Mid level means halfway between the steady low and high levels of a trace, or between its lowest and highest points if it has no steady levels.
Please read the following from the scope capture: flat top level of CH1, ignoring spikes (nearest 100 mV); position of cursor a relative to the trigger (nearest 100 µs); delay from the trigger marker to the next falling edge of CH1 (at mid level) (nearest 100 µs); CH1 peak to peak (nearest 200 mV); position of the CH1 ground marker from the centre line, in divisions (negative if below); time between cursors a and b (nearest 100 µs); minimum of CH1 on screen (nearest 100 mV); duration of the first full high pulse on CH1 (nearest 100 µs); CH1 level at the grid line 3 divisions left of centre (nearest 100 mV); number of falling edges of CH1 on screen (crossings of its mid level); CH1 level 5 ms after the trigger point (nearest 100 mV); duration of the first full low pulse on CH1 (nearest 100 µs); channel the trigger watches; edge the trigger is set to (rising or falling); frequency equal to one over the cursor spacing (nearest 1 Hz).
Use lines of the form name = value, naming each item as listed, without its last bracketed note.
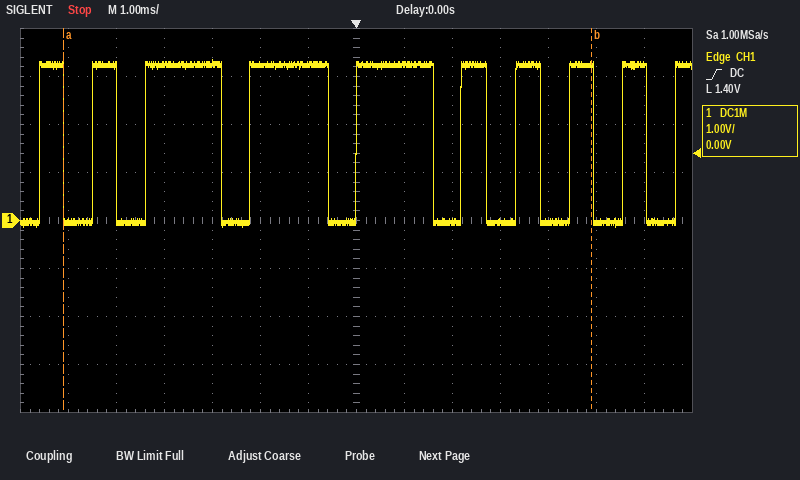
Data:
flat top level of CH1, ignoring spikes = 3.2 V
position of cursor a relative to the trigger = -6.1 ms
delay from the trigger marker to the next falling edge of CH1 (at mid level) = 1.6 ms
CH1 peak to peak = 3.4 V
position of the CH1 ground marker from the centre line, in divisions = 0.0 div
time between cursors a and b = 11.0 ms
minimum of CH1 on screen = -100 mV
duration of the first full high pulse on CH1 = 500 µs
CH1 level at the grid line 3 divisions left of centre = 3.3 V
number of falling edges of CH1 on screen = 9
CH1 level 5 ms after the trigger point = 0.0 V
duration of the first full low pulse on CH1 = 600 µs
channel the trigger watches = CH1
edge the trigger is set to = rising
frequency equal to one over the cursor spacing = 91 Hz
